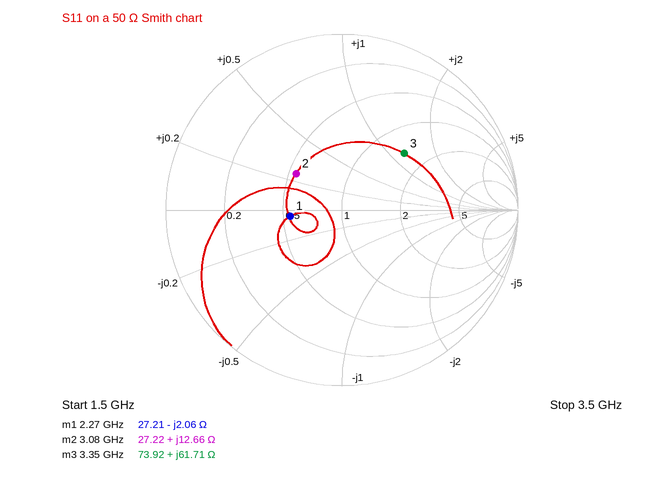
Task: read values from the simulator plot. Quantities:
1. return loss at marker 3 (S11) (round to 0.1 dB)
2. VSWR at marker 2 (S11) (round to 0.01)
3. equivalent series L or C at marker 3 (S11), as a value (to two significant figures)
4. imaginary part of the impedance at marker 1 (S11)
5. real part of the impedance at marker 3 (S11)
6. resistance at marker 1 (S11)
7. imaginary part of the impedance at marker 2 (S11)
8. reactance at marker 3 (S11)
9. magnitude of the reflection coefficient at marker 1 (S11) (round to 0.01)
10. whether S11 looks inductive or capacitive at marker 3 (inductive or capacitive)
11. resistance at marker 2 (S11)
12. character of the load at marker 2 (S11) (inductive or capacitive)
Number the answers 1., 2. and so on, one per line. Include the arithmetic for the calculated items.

1. 6.4 dB
2. 2.00
3. L = 61.71 Ω/(2π × 3.35 GHz) ≈ 2.9 nH
4. -2.06 Ω
5. 73.92 Ω
6. 27.21 Ω
7. +12.66 Ω
8. +61.71 Ω
9. 0.30
10. inductive
11. 27.22 Ω
12. inductive
